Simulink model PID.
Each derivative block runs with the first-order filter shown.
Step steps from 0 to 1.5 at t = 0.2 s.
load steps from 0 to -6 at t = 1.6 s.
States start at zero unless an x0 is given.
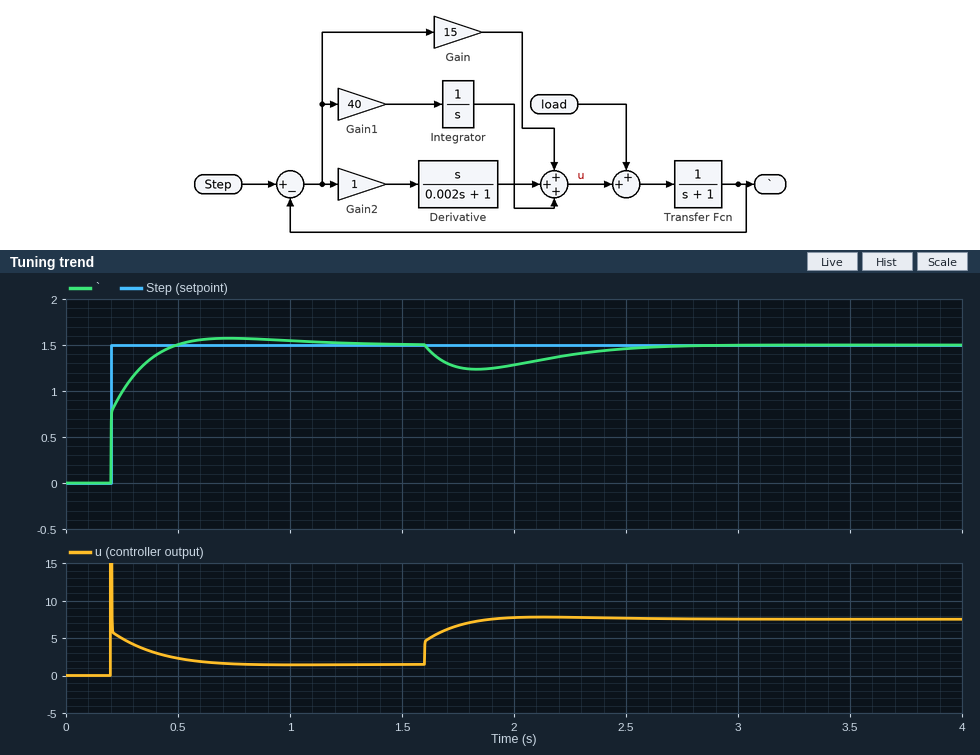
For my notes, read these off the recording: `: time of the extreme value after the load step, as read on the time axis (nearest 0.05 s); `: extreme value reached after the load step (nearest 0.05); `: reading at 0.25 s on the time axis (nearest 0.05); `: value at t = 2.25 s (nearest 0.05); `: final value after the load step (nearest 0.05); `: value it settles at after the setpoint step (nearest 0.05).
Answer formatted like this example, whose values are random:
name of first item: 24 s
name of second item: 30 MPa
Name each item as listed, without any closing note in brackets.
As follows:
`: time of the extreme value after the load step, as read on the time axis: 1.85 s
`: extreme value reached after the load step: 1.25
`: reading at 0.25 s on the time axis: 1.00
`: value at t = 2.25 s: 1.40
`: final value after the load step: 1.50
`: value it settles at after the setpoint step: 1.50
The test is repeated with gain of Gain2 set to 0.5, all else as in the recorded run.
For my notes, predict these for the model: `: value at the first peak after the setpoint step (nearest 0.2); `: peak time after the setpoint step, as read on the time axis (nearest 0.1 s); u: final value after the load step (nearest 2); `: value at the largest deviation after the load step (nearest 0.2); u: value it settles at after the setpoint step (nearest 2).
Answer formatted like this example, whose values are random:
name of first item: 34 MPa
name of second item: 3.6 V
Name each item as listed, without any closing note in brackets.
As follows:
`: value at the first peak after the setpoint step: 1.6
`: peak time after the setpoint step, as read on the time axis: 0.6 s
u: final value after the load step: 8
`: value at the largest deviation after the load step: 1.2
u: value it settles at after the setpoint step: 2
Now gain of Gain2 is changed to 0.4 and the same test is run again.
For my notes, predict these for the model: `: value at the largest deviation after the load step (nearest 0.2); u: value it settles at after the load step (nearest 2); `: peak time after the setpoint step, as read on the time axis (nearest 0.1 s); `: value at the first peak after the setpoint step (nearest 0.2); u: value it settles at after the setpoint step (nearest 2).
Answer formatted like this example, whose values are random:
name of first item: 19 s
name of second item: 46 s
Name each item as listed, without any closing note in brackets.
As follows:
`: value at the largest deviation after the load step: 1.2
u: value it settles at after the load step: 8
`: peak time after the setpoint step, as read on the time axis: 0.6 s
`: value at the first peak after the setpoint step: 1.6
u: value it settles at after the setpoint step: 2
